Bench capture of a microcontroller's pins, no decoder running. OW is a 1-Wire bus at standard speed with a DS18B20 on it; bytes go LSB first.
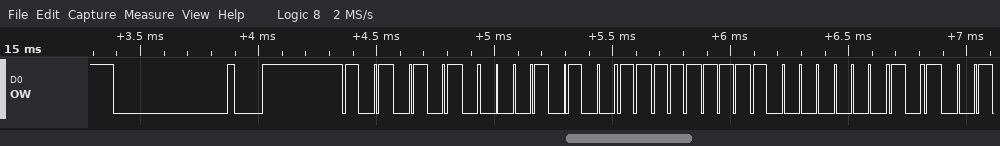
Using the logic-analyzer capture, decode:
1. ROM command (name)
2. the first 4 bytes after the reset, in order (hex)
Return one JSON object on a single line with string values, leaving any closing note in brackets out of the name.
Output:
{"ROM command": "Match ROM", "the first 4 bytes after the reset, in order": "55 28 FF 01"}
